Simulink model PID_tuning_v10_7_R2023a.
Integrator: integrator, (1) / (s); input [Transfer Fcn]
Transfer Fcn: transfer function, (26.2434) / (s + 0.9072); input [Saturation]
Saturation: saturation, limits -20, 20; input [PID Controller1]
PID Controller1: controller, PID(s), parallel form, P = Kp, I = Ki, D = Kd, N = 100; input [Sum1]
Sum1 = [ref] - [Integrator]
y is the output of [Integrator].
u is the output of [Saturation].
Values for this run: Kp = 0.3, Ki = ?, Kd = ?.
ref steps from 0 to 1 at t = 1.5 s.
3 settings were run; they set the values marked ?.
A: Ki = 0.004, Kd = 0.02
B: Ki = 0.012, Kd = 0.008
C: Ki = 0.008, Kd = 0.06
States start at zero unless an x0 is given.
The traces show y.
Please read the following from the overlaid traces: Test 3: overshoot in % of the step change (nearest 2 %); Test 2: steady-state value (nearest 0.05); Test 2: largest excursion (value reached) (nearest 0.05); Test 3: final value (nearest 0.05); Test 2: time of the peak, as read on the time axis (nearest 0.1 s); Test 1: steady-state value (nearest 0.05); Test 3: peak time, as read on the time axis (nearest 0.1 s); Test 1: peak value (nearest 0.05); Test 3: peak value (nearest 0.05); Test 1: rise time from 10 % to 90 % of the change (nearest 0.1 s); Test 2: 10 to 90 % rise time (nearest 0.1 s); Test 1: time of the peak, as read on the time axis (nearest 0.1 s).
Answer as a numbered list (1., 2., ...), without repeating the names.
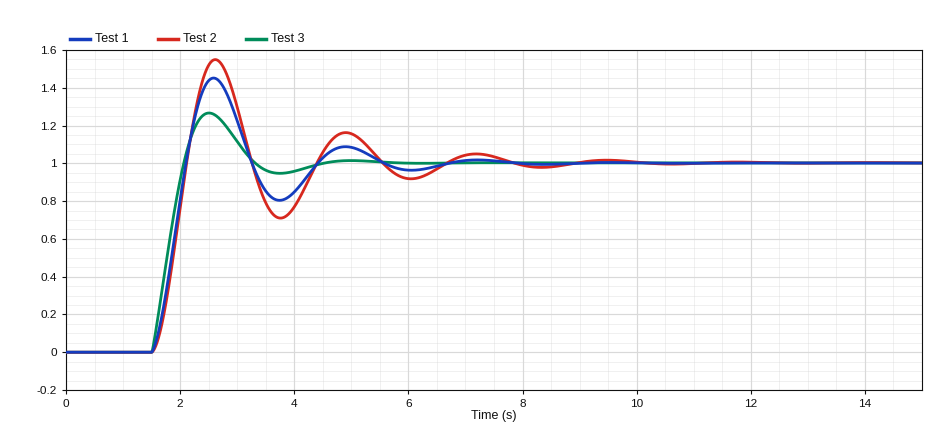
1. 26 %
2. 1.00
3. 1.55
4. 1.00
5. 2.6 s
6. 1.00
7. 2.5 s
8. 1.45
9. 1.25
10. 0.4 s
11. 0.4 s
12. 2.6 s
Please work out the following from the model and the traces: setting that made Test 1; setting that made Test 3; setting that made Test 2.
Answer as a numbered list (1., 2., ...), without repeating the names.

1. A
2. C
3. B
